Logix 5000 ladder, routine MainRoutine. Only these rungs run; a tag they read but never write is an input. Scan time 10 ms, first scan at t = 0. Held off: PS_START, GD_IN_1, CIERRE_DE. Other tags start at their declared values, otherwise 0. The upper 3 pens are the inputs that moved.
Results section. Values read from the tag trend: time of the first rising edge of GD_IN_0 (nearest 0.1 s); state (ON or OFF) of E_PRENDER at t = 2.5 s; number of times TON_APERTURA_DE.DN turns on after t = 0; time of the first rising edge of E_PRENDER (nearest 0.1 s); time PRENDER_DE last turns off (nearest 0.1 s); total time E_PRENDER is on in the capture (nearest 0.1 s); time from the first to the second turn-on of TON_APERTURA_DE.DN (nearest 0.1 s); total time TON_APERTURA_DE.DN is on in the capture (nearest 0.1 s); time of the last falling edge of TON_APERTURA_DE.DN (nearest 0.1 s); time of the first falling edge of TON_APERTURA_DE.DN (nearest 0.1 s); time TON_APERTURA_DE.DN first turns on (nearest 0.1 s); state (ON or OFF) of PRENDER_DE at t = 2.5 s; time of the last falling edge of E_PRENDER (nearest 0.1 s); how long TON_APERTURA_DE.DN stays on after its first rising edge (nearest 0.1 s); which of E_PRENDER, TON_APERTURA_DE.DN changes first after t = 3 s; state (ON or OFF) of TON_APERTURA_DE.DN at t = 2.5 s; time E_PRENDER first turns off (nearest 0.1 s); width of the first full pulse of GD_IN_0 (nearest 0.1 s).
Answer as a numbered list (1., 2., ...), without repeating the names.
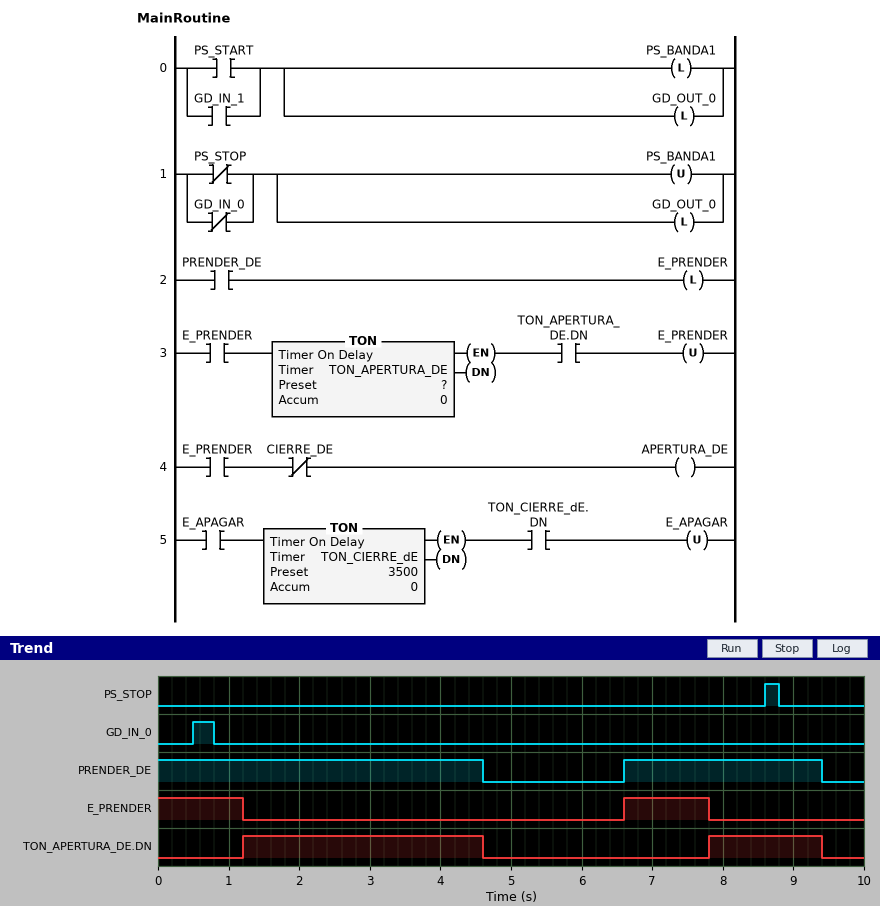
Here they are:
1. 0.5 s
2. OFF
3. 2
4. 6.6 s
5. 9.4 s
6. 2.4 s
7. 6.6 s
8. 5.0 s
9. 9.4 s
10. 4.6 s
11. 1.2 s
12. ON
13. 7.8 s
14. 3.4 s
15. TON_APERTURA_DE.DN
16. ON
17. 1.2 s
18. 0.3 s
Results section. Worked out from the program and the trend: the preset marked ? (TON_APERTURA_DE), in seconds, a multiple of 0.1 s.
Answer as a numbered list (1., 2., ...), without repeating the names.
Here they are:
1. 1.2 s
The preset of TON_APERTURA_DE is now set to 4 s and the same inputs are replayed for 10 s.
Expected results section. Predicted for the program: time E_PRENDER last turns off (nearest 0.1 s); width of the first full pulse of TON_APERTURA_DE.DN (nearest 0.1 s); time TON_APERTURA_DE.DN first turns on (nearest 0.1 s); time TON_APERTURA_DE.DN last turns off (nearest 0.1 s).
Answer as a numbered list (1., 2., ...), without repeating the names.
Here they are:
1. 4.0 s
2. 0.6 s
3. 4.0 s
4. 4.6 s
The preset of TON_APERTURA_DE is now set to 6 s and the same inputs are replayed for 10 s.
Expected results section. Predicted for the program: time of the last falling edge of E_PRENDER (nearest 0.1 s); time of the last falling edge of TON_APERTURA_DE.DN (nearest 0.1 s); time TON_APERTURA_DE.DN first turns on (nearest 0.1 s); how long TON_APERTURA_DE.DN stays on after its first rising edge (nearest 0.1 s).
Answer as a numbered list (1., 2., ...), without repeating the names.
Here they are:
1. 6.0 s
2. 6.0 s
3. 6.0 s
4. 0.0 s
